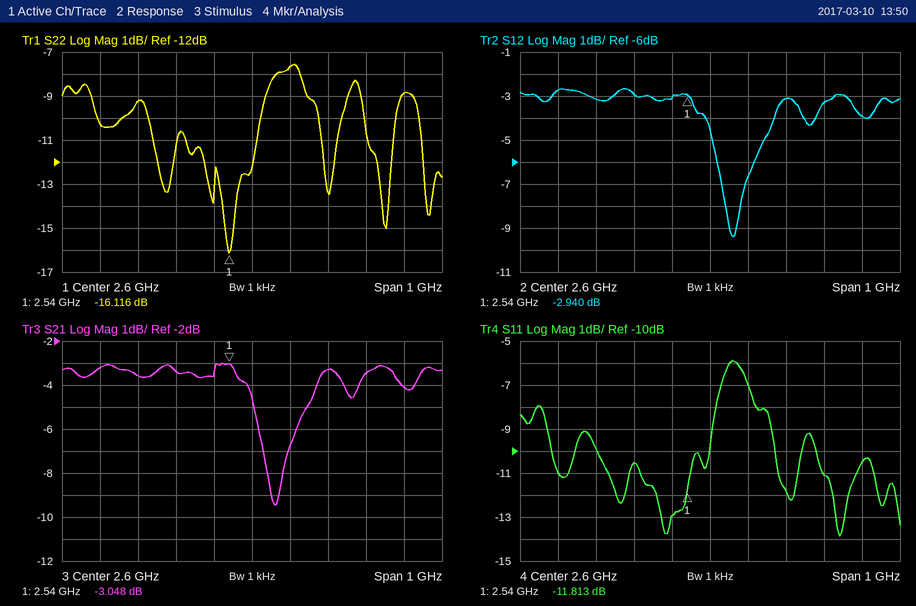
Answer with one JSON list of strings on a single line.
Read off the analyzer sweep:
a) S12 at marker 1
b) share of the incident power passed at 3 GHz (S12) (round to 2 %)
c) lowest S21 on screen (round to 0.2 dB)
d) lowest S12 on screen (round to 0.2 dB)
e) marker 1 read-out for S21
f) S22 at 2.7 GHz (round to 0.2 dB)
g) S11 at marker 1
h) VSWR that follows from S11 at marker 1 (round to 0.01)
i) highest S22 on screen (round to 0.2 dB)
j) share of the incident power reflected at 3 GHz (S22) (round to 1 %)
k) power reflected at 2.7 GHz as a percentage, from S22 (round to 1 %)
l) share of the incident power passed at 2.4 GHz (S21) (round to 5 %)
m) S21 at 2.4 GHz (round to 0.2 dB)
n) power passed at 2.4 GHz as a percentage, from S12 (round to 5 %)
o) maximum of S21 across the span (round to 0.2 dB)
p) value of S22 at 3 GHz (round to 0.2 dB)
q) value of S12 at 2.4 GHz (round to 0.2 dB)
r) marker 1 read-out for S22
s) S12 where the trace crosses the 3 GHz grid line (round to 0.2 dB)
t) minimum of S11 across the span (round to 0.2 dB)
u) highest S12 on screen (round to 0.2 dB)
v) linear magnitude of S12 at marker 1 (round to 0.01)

["-2.940 dB", "40 %", "-9.4 dB", "-9.4 dB", "-3.048 dB", "-7.6 dB", "-11.813 dB", "1.69", "-7.6 dB", "13 %", "17 %", "45 %", "-3.4 dB", "50 %", "-3.0 dB", "-8.8 dB", "-3.0 dB", "-16.116 dB", "-4.0 dB", "-13.8 dB", "-2.6 dB", "0.71"]
